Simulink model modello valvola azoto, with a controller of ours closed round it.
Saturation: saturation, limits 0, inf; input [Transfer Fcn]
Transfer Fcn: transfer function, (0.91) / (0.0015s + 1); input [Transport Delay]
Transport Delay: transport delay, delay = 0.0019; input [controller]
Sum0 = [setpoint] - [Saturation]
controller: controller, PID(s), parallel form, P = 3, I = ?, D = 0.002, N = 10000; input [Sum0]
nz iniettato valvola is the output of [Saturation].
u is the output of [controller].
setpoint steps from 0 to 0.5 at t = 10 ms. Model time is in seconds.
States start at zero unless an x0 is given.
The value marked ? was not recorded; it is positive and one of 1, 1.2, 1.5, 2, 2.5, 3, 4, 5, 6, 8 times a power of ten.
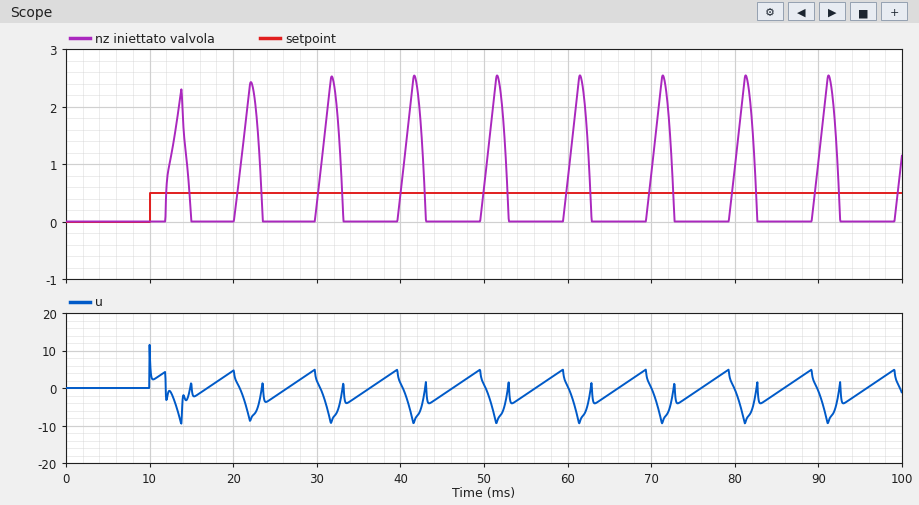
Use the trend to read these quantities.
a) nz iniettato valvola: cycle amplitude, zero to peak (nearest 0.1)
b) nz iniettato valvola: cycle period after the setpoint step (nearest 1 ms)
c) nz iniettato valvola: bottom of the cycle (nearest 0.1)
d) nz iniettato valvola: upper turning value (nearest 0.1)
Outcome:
1.3
10 ms
0.0
2.5
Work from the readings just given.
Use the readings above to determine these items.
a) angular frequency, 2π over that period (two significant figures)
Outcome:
0.63 rad/ms
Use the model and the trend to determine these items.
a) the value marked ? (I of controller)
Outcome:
3000
